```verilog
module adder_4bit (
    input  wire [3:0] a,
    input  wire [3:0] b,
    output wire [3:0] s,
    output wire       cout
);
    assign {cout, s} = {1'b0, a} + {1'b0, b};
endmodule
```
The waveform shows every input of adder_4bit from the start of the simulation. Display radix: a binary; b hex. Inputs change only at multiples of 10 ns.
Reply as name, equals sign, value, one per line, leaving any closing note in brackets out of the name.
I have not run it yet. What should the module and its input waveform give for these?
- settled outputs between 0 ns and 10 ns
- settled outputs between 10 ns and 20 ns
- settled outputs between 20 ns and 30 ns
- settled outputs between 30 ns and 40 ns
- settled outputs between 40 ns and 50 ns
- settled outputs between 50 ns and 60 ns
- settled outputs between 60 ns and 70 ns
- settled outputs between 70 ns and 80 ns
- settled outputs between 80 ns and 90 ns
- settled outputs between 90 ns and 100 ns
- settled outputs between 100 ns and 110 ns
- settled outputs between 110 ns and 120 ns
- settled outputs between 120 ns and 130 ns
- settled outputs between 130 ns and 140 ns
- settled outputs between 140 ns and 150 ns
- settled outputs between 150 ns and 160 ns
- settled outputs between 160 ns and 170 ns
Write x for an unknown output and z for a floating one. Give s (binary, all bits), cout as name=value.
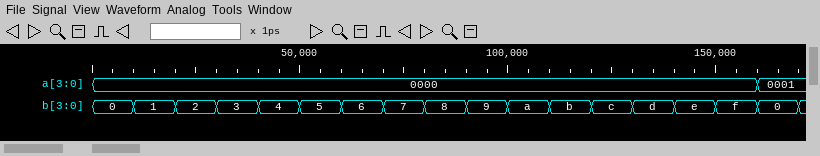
settled outputs between 0 ns and 10 ns = s=0000, cout=0
settled outputs between 10 ns and 20 ns = s=0001, cout=0
settled outputs between 20 ns and 30 ns = s=0010, cout=0
settled outputs between 30 ns and 40 ns = s=0011, cout=0
settled outputs between 40 ns and 50 ns = s=0100, cout=0
settled outputs between 50 ns and 60 ns = s=0101, cout=0
settled outputs between 60 ns and 70 ns = s=0110, cout=0
settled outputs between 70 ns and 80 ns = s=0111, cout=0
settled outputs between 80 ns and 90 ns = s=1000, cout=0
settled outputs between 90 ns and 100 ns = s=1001, cout=0
settled outputs between 100 ns and 110 ns = s=1010, cout=0
settled outputs between 110 ns and 120 ns = s=1011, cout=0
settled outputs between 120 ns and 130 ns = s=1100, cout=0
settled outputs between 130 ns and 140 ns = s=1101, cout=0
settled outputs between 140 ns and 150 ns = s=1110, cout=0
settled outputs between 150 ns and 160 ns = s=1111, cout=0
settled outputs between 160 ns and 170 ns = s=0001, cout=0
